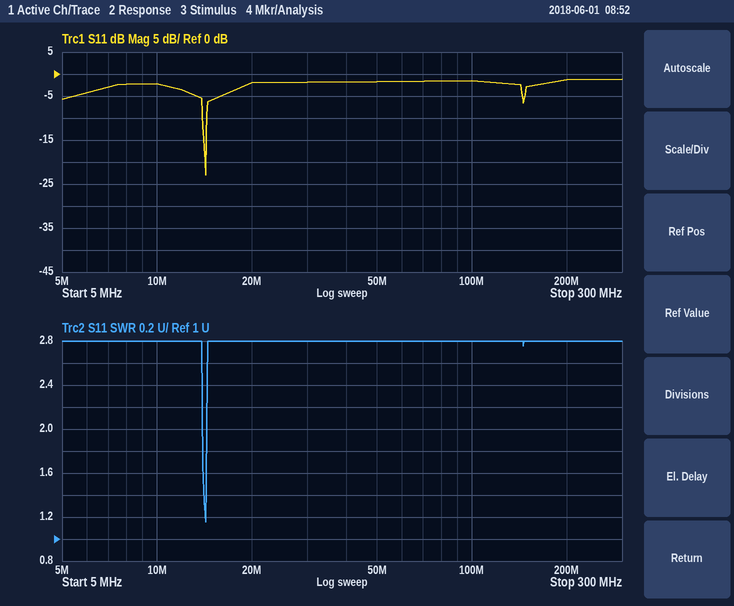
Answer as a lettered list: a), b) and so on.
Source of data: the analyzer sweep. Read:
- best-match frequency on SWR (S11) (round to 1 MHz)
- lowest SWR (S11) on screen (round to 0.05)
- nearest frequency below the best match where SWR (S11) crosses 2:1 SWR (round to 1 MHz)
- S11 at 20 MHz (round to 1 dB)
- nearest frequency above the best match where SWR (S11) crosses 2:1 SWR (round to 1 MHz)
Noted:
a) 14 MHz
b) 1.15
c) 14 MHz
d) -2 dB
e) 14 MHz
